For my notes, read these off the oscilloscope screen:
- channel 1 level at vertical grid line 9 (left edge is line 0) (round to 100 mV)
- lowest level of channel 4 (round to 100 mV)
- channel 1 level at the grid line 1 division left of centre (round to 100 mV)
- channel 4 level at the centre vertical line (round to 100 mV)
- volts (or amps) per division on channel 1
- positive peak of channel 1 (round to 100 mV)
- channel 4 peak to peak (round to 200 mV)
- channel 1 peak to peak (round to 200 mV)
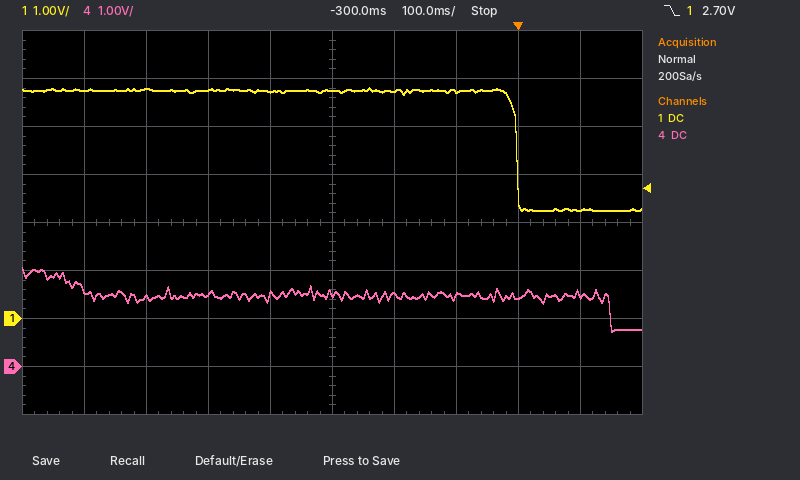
2.3 V
700 mV
4.7 V
1.5 V
1 V
4.8 V
1.4 V
2.6 V
